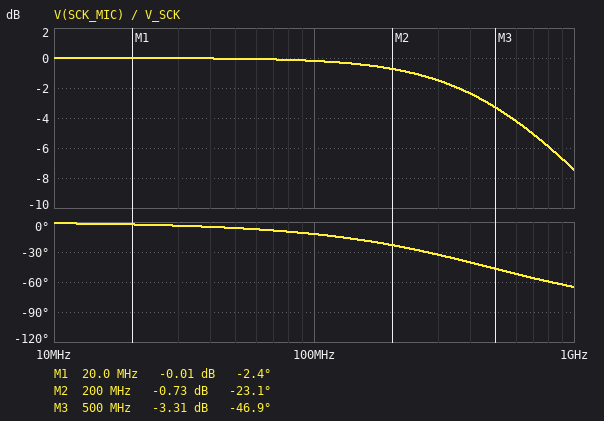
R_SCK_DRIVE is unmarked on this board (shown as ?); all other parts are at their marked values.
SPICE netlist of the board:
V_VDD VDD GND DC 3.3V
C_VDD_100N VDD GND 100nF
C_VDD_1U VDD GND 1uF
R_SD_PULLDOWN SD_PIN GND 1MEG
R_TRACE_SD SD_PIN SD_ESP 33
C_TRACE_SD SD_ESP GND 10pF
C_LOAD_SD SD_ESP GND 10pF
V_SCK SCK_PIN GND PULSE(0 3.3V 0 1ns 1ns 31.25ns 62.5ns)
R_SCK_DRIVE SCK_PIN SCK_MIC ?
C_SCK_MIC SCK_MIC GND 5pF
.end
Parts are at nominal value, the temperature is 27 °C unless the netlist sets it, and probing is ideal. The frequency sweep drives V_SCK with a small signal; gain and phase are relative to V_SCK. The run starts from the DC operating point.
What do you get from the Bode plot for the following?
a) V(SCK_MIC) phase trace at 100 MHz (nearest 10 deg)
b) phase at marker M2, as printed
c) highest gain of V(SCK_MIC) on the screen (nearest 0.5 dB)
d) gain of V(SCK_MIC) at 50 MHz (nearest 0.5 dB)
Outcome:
-10 deg
-23.1 deg
0 dB
0 dB
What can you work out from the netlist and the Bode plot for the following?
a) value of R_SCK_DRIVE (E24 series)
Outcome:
68 Ω
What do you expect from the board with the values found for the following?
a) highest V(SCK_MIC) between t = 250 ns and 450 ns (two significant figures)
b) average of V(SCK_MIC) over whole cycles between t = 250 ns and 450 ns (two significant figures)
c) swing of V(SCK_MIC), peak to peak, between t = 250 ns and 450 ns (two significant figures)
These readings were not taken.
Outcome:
3.3 V
1.7 V
3.3 V
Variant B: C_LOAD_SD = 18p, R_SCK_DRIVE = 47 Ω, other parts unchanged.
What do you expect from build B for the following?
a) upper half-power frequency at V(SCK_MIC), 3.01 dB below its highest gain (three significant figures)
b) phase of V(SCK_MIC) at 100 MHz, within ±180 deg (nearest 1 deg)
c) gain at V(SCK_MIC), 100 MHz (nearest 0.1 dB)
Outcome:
677 MHz
-8 deg
-0.1 dB
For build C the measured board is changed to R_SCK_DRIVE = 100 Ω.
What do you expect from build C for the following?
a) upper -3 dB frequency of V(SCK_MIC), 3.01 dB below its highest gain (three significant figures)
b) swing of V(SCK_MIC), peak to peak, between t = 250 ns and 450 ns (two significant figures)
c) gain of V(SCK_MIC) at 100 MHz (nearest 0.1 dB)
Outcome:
318 MHz
3.3 V
-0.4 dB
